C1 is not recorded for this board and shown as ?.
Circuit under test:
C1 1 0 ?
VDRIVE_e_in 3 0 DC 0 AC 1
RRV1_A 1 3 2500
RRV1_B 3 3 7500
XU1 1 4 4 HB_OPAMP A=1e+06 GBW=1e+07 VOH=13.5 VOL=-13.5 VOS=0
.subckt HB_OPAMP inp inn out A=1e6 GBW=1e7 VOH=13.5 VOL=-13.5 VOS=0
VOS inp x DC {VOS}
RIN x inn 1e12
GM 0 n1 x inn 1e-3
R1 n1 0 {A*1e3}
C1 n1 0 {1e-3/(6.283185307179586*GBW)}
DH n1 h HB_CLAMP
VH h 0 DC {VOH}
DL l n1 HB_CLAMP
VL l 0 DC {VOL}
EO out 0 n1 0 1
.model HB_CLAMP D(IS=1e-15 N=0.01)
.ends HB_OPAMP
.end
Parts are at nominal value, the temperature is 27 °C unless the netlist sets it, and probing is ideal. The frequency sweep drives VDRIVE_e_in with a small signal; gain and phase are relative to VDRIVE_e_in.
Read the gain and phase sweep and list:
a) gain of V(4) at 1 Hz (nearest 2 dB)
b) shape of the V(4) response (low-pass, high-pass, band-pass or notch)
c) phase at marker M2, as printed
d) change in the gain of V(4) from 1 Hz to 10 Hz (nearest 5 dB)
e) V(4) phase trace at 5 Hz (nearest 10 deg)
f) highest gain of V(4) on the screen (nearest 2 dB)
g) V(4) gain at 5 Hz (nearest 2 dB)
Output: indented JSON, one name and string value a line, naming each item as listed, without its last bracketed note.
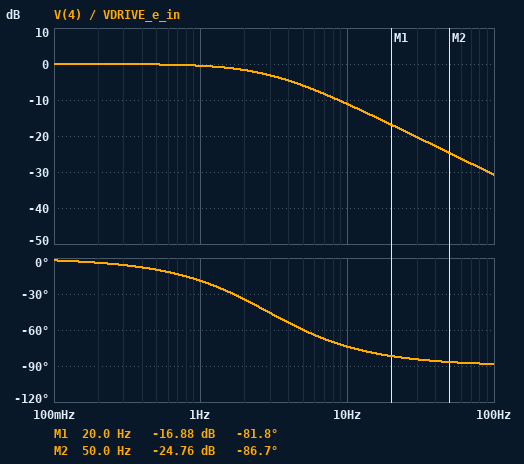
{
  "gain of V(4) at 1 Hz": "0 dB",
  "shape of the V(4) response": "low-pass",
  "phase at marker M2, as printed": "-86.7 deg",
  "change in the gain of V(4) from 1 Hz to 10 Hz": "-10 dB",
  "V(4) phase trace at 5 Hz": "-60 deg",
  "highest gain of V(4) on the screen": "0 dB",
  "V(4) gain at 5 Hz": "-6 dB"
}
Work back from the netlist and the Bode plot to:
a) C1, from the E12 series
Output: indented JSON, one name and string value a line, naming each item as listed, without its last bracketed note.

{
  "C1, from the E12 series": "22 µF"
}
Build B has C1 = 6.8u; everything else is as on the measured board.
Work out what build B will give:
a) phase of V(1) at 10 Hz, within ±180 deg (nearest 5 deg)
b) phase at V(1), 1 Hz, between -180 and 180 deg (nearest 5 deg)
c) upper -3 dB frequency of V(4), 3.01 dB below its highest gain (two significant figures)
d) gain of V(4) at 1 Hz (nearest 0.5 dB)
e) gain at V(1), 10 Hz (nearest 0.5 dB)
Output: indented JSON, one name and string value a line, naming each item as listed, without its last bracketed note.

{
  "phase of V(1) at 10 Hz, within ±180 deg": "-45 deg",
  "phase at V(1), 1 Hz, between -180 and 180 deg": "-5 deg",
  "upper -3 dB frequency of V(4), 3.01 dB below its highest gain": "9.4 Hz",
  "gain of V(4) at 1 Hz": "0 dB",
  "gain at V(1), 10 Hz": "-3.5 dB"
}
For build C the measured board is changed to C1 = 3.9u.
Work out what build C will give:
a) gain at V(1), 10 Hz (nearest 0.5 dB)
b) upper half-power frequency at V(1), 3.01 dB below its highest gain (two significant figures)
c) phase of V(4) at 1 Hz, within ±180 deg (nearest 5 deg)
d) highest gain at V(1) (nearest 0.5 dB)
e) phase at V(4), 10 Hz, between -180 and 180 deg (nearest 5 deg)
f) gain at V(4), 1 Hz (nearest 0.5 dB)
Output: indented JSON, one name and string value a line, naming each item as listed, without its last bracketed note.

{
  "gain at V(1), 10 Hz": "-1.5 dB",
  "upper half-power frequency at V(1), 3.01 dB below its highest gain": "16 Hz",
  "phase of V(4) at 1 Hz, within ±180 deg": "-5 deg",
  "highest gain at V(1)": "0 dB",
  "phase at V(4), 10 Hz, between -180 and 180 deg": "-30 deg",
  "gain at V(4), 1 Hz": "0 dB"
}
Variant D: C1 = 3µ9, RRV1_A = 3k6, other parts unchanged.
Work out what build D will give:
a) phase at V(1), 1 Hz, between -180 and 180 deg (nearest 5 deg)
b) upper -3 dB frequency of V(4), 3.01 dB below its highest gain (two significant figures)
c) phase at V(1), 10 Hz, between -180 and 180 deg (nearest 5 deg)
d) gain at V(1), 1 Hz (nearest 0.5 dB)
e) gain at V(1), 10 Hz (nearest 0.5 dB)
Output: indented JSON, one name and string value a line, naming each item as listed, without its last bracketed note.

{
  "phase at V(1), 1 Hz, between -180 and 180 deg": "-5 deg",
  "upper -3 dB frequency of V(4), 3.01 dB below its highest gain": "11 Hz",
  "phase at V(1), 10 Hz, between -180 and 180 deg": "-40 deg",
  "gain at V(1), 1 Hz": "0 dB",
  "gain at V(1), 10 Hz": "-2.5 dB"
}
